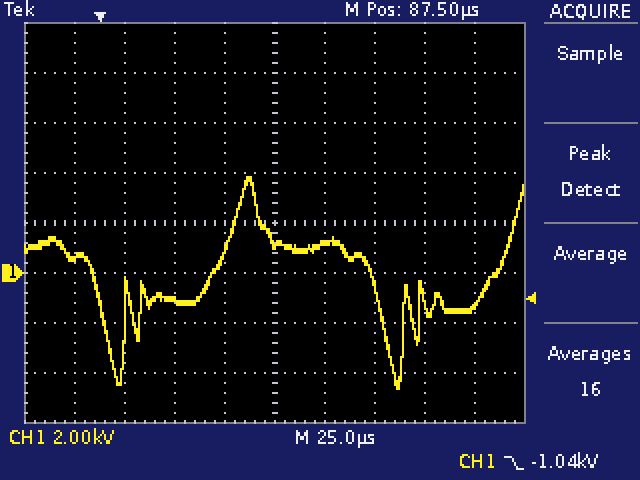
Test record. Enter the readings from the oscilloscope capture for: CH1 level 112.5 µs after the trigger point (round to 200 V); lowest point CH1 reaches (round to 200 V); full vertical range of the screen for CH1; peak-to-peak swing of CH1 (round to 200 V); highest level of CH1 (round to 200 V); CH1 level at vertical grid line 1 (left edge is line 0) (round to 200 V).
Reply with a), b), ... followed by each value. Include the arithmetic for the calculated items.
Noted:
a) 1.2 kV
b) -4.6 kV
c) 16 kV
d) 3.8 kV − (-4.6 kV) = 8.4 kV
e) 3.8 kV
f) 600 V
